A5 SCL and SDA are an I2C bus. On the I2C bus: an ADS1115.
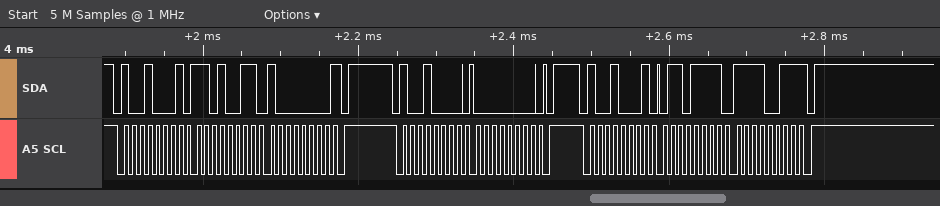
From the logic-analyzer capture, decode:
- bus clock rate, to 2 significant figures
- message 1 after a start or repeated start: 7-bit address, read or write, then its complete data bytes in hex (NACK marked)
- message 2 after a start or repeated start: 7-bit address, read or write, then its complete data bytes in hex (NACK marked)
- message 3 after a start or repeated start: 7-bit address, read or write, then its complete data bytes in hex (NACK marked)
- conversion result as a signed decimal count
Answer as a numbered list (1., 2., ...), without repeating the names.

1. 100 kHz
2. 0x48 read: D3 80 NACK
3. 0x48 write: 00
4. 0x48 read: 6F F3 NACK
5. 28659
